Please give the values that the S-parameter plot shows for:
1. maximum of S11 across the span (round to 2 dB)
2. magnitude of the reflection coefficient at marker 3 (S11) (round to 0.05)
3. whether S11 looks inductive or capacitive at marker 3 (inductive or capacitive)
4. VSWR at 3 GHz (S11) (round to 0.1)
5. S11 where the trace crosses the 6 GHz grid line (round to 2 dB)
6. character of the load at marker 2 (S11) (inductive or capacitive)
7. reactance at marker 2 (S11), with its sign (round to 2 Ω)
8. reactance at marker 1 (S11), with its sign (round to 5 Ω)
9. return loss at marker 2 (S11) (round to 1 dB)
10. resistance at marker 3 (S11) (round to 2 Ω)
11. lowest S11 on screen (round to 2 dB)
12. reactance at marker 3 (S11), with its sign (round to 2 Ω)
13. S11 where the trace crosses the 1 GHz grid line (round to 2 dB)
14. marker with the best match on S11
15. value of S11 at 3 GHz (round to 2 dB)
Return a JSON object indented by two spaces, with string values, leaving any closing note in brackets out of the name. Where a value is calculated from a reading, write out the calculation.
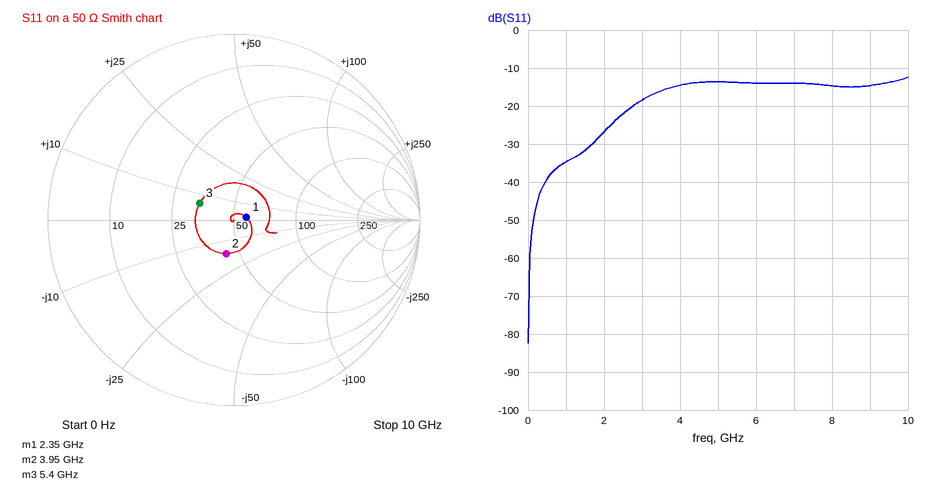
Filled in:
{
  "maximum of S11 across the span": "-12 dB",
  "magnitude of the reflection coefficient at marker 3 (S11)": "0.20",
  "whether S11 looks inductive or capacitive at marker 3": "inductive",
  "VSWR at 3 GHz (S11)": "|Γ| = 10^(-18/20) = 0.1259; VSWR = (1 + 0.1259)/(1 − 0.1259) ≈ 1.3",
  "S11 where the trace crosses the 6 GHz grid line": "-14 dB",
  "character of the load at marker 2 (S11)": "capacitive",
  "reactance at marker 2 (S11), with its sign": "-16 Ω",
  "reactance at marker 1 (S11), with its sign": "0 Ω",
  "return loss at marker 2 (S11)": "15 dB",
  "resistance at marker 3 (S11)": "34 Ω",
  "lowest S11 on screen": "-82 dB",
  "reactance at marker 3 (S11), with its sign": "+6 Ω",
  "S11 where the trace crosses the 1 GHz grid line": "-34 dB",
  "marker with the best match on S11": "marker 1",
  "value of S11 at 3 GHz": "-18 dB"
}
